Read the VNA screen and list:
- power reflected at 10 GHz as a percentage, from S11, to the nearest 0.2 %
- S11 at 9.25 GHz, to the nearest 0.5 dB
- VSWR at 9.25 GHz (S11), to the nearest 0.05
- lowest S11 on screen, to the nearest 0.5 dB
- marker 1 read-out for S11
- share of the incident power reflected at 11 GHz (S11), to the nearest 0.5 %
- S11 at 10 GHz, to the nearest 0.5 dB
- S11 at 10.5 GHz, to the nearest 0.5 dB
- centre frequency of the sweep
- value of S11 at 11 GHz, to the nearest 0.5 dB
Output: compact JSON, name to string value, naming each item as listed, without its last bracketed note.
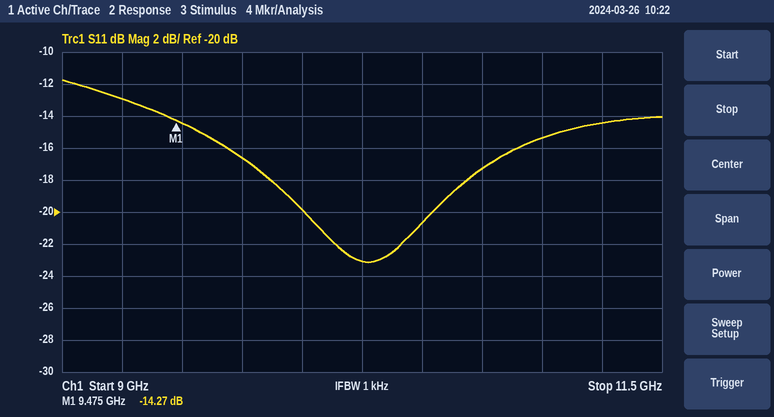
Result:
{"power reflected at 10 GHz as a percentage, from S11, to the nearest 0.2 %": "1.0 %", "S11 at 9.25 GHz, to the nearest 0.5 dB": "-13.0 dB", "VSWR at 9.25 GHz (S11), to the nearest 0.05": "1.60", "lowest S11 on screen, to the nearest 0.5 dB": "-23.0 dB", "marker 1 read-out for S11": "-14.27 dB", "share of the incident power reflected at 11 GHz (S11), to the nearest 0.5 %": "3.0 %", "S11 at 10 GHz, to the nearest 0.5 dB": "-20.0 dB", "S11 at 10.5 GHz, to the nearest 0.5 dB": "-20.5 dB", "centre frequency of the sweep": "10.25 GHz", "value of S11 at 11 GHz, to the nearest 0.5 dB": "-15.5 dB"}
